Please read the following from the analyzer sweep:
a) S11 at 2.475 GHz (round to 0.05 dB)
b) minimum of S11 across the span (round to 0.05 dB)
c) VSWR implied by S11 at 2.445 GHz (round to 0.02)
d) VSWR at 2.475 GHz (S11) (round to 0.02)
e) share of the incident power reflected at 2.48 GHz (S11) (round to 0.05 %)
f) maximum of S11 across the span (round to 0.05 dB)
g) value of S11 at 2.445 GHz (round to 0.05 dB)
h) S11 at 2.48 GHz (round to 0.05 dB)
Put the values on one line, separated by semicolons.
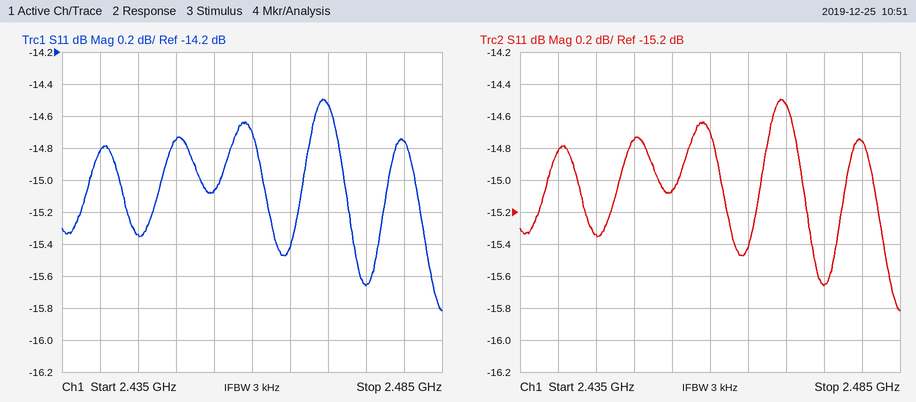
-15.65 dB; -15.80 dB; 1.42; 1.40; 3.35 %; -14.50 dB; -15.35 dB; -14.75 dB
